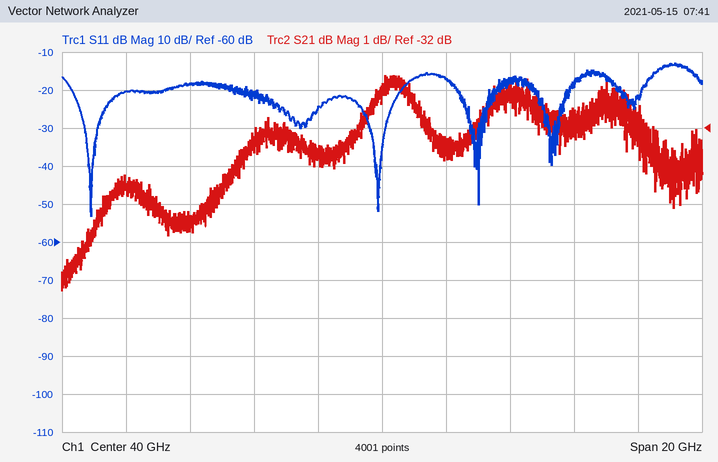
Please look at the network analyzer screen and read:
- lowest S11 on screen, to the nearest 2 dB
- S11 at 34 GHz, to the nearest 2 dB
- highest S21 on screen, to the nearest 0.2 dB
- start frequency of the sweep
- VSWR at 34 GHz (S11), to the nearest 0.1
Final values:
-54 dB
-18 dB
-30.6 dB
30 GHz
1.3
